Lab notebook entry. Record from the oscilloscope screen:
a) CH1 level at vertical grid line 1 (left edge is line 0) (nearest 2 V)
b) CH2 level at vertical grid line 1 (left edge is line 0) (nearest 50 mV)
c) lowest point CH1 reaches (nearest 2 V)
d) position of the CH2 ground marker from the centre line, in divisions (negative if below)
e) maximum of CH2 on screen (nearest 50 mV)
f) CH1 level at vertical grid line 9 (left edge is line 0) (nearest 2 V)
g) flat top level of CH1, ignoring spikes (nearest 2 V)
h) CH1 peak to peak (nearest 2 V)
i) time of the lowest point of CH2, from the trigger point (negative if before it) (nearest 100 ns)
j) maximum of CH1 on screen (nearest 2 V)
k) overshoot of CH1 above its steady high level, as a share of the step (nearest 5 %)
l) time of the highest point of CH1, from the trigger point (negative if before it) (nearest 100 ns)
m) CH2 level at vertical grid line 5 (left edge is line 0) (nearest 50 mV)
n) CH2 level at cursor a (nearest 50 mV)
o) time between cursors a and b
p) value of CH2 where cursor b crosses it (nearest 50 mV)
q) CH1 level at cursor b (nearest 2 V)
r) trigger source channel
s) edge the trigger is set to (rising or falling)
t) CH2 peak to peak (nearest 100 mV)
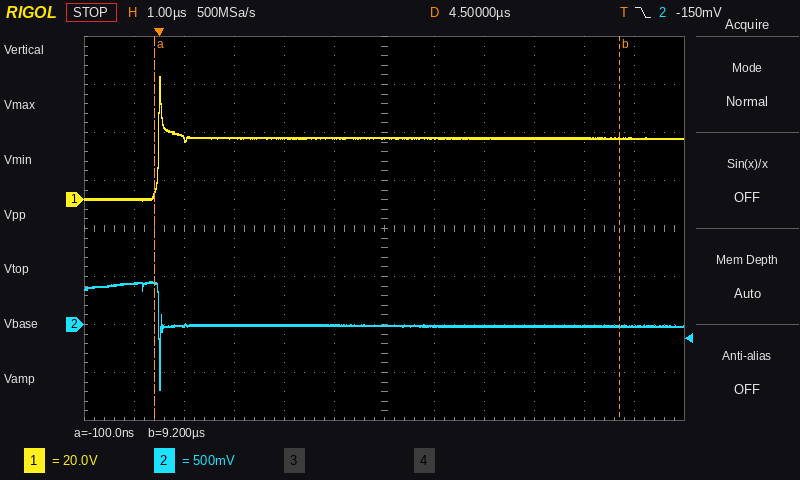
0 V
450 mV
0 V
-2.0 div
450 mV
26 V
26 V
52 V
0.0 µs
52 V
100 %
0.0 µs
0 mV
400 mV
9.3 µs
0 mV
26 V
CH2
falling
1.10 V
